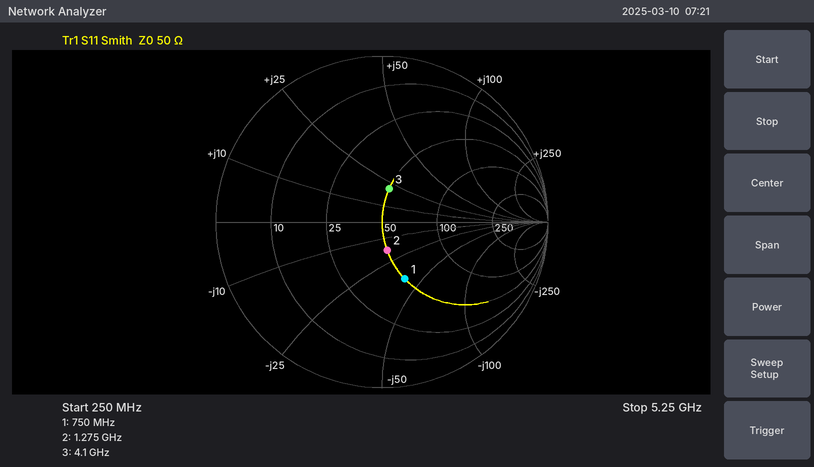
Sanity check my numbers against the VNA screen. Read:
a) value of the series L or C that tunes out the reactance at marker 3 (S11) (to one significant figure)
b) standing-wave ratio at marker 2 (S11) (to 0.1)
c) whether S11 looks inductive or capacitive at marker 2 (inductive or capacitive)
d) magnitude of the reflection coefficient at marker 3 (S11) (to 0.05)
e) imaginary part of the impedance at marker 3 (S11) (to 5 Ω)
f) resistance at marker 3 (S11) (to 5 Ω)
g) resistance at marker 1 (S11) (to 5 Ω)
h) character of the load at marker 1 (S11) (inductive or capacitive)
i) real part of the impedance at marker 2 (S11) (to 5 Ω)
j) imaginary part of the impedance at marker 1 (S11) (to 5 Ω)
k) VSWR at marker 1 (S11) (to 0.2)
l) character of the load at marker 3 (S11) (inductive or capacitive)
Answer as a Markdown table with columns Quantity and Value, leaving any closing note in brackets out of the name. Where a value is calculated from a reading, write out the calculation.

| Quantity | Value |
|---|---|
| value of the series L or C that tunes out the reactance at marker 3 (S11) | C = 1/(2π × 4.1 GHz × 20 Ω) ≈ 2 pF |
| standing-wave ratio at marker 2 (S11) | 1.4 |
| whether S11 looks inductive or capacitive at marker 2 | capacitive |
| magnitude of the reflection coefficient at marker 3 (S11) | 0.20 |
| imaginary part of the impedance at marker 3 (S11) | +20 Ω |
| resistance at marker 3 (S11) | 50 Ω |
| resistance at marker 1 (S11) | 50 Ω |
| character of the load at marker 1 (S11) | capacitive |
| real part of the impedance at marker 2 (S11) | 50 Ω |
| imaginary part of the impedance at marker 1 (S11) | -40 Ω |
| VSWR at marker 1 (S11) | 2.2 |
| character of the load at marker 3 (S11) | inductive |
